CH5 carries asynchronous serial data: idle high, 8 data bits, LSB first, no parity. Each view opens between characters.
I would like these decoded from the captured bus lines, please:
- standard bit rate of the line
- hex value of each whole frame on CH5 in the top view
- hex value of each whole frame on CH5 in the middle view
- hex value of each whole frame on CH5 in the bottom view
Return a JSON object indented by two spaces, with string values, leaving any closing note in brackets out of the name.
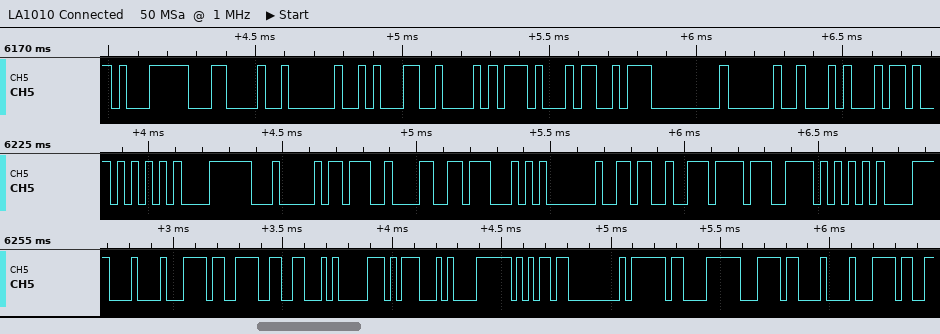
{
  "standard bit rate of the line": "38400 baud",
  "hex value of each whole frame on CH5 in the top view": "F1, 0C, 02, 8A, 42, 17, D3, 00, 20, 14",
  "hex value of each whole frame on CH5 in the middle view": "55, F8, 04, 3B, 98, 47, 01, 36, EE, E7, 55",
  "hex value of each whole frame on CH5 in the bottom view": "08, BC, 9E, 46, 70, 47, F8, B5, 00, BF, F8, BC, 08, BC"
}
